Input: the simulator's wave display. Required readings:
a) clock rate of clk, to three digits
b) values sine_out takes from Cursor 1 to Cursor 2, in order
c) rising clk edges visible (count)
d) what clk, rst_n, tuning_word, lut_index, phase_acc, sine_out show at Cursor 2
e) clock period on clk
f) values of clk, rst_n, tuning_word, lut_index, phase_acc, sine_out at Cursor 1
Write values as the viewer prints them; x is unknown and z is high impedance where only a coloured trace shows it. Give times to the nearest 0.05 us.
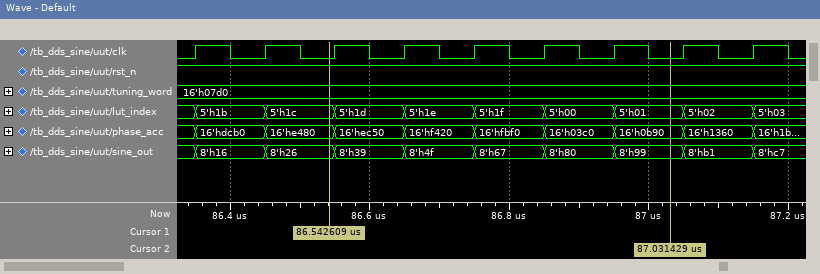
10.0 MHz
8'h26, 8'h39, 8'h4f, 8'h67, 8'h80, 8'h99
9
clk=0, rst_n=1, tuning_word=16'h07d0, lut_index=5'h01, phase_acc=16'h0b90, sine_out=8'h99
0.1 us
clk=0, rst_n=1, tuning_word=16'h07d0, lut_index=5'h1c, phase_acc=16'he480, sine_out=8'h26
